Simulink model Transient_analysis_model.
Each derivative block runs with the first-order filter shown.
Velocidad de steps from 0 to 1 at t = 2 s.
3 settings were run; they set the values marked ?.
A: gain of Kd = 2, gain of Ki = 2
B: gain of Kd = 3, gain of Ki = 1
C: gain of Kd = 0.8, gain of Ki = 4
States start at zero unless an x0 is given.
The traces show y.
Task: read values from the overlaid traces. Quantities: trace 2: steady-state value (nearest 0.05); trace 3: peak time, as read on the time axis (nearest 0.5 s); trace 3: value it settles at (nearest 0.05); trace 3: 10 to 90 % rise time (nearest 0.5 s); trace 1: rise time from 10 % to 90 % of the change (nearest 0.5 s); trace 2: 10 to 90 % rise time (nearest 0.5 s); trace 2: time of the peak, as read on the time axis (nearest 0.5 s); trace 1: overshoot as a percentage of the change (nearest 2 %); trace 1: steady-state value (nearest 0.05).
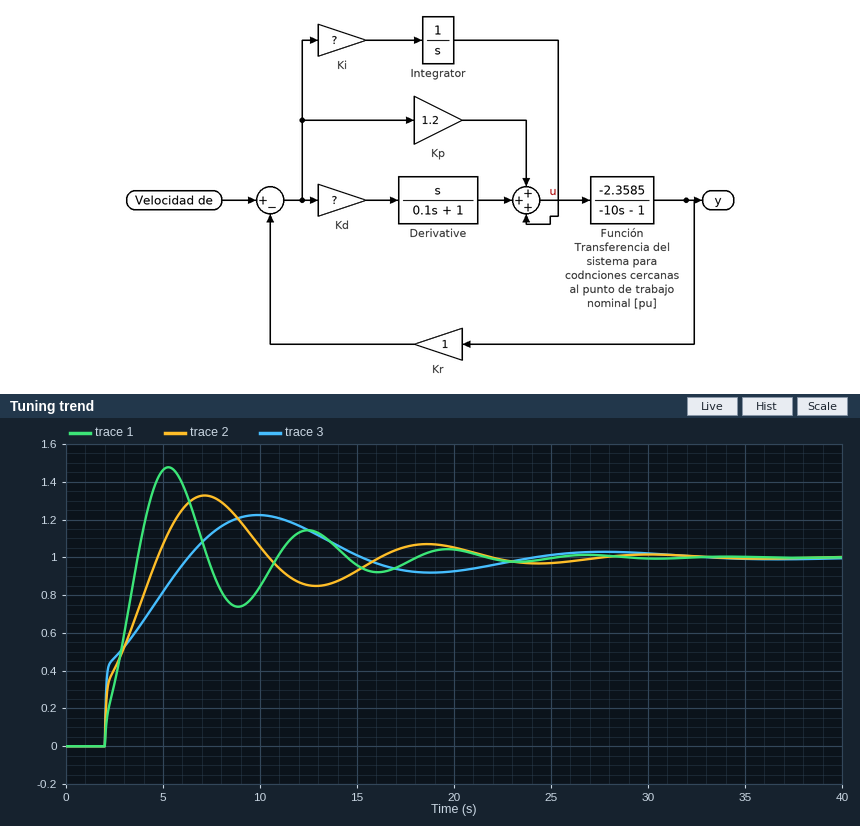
1.00
10.0 s
1.00
3.5 s
1.5 s
2.5 s
7.0 s
48 %
1.00
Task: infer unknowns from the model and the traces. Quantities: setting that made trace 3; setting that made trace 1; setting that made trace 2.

B
C
A
